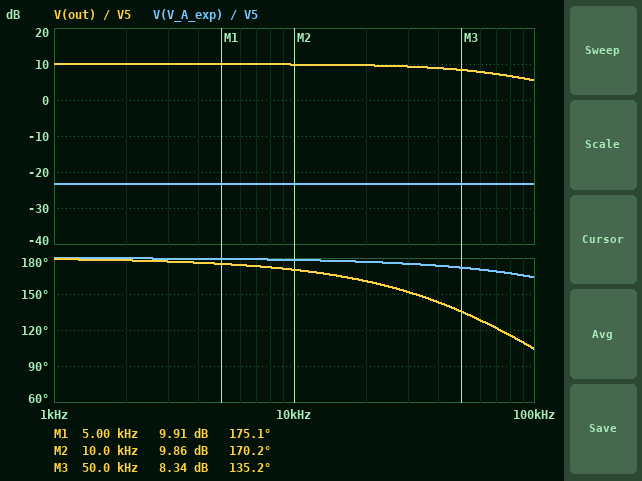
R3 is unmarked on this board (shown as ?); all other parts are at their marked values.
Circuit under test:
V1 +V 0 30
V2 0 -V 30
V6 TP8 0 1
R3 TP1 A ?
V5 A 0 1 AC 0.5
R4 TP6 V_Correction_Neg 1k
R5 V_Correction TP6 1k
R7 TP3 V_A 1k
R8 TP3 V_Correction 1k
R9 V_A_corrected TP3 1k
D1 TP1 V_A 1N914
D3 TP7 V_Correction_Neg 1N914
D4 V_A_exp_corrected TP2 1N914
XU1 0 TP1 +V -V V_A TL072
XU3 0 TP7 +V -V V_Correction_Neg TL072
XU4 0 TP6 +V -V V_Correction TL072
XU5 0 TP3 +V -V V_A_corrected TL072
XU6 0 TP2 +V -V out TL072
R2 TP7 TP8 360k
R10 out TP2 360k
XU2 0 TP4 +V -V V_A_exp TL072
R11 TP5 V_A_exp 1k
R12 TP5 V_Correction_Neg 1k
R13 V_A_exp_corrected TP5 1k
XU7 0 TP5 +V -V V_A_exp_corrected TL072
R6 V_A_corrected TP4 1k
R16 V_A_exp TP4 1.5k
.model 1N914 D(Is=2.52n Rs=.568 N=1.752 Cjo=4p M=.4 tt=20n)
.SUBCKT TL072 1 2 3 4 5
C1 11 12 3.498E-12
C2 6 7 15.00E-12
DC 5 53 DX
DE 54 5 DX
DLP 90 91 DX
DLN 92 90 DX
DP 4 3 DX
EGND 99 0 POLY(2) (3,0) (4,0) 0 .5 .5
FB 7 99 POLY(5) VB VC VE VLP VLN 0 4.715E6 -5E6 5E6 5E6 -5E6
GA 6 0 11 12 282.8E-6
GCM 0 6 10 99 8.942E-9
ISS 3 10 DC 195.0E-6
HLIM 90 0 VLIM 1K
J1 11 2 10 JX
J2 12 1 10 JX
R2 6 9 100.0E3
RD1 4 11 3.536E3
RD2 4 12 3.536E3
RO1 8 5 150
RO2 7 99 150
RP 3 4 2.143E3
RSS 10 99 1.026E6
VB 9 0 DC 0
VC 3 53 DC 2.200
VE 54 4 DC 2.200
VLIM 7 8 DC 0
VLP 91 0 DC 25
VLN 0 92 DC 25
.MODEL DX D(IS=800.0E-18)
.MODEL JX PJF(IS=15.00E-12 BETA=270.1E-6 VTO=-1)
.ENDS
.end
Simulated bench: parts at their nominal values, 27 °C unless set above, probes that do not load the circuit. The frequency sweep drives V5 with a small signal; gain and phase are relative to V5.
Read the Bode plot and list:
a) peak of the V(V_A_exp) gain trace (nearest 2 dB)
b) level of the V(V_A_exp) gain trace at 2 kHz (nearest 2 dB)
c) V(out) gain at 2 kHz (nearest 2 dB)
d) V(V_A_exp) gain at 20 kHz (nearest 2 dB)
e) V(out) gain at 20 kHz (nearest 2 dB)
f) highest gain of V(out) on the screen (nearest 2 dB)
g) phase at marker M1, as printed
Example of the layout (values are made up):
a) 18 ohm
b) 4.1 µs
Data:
a) -24 dB
b) -24 dB
c) 10 dB
d) -24 dB
e) 10 dB
f) 10 dB
g) 175.1 deg
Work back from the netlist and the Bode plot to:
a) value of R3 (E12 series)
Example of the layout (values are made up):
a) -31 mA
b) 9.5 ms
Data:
a) 220 kΩ
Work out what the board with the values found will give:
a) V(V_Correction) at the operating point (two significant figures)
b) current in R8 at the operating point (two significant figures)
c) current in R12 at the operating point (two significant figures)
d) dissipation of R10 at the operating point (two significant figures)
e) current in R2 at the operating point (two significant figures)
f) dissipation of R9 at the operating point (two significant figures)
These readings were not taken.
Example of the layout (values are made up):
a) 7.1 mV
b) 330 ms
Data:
a) 320 mV
b) 320 µA
c) 320 µA
d) 12 µW
e) 2.8 µA
f) 500 nW
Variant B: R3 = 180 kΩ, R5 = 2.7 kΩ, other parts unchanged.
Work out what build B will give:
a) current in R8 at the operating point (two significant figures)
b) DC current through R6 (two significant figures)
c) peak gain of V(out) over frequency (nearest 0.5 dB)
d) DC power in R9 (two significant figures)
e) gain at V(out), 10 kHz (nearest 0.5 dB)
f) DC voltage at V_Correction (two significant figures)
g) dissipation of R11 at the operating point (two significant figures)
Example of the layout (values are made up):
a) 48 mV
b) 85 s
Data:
a) 860 µA
b) 510 µA
c) 8.0 dB
d) 260 µW
e) -45.5 dB
f) 860 mV
g) 580 µW
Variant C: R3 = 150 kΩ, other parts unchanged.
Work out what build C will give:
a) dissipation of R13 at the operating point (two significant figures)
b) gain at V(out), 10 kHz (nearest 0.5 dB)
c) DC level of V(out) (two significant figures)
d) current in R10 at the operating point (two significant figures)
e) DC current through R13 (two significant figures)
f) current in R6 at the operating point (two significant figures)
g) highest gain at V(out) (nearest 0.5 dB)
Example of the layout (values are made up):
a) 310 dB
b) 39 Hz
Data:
a) 140 µW
b) 14.5 dB
c) -3.7 V
d) 10 µA
e) 380 µA
f) 40 µA
g) 15.0 dB
